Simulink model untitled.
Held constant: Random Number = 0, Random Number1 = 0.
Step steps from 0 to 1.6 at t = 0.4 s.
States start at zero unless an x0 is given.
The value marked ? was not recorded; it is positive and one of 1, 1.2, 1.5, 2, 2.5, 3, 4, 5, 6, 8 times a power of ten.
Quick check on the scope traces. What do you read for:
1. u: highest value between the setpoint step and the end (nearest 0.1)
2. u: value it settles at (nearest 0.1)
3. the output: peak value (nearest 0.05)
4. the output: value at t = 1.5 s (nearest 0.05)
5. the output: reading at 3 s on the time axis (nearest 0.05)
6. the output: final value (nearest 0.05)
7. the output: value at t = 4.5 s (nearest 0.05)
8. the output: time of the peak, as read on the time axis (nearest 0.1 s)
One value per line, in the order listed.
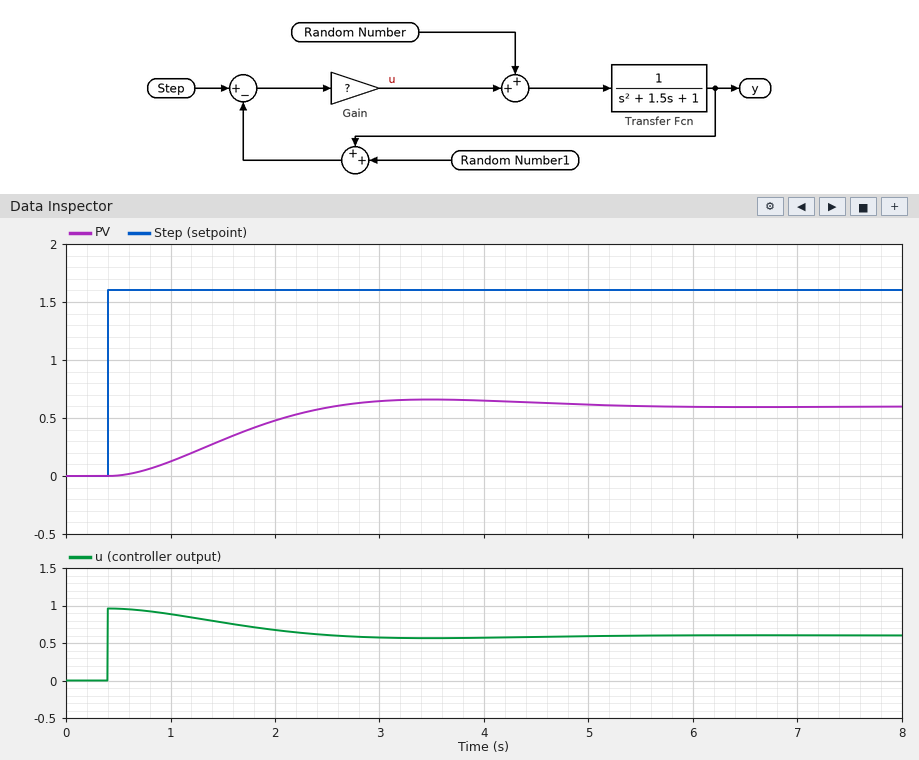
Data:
1.0
0.6
0.65
0.30
0.65
0.60
0.65
3.5 s
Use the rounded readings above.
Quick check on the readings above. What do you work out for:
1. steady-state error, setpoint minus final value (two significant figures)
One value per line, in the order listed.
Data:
1.0
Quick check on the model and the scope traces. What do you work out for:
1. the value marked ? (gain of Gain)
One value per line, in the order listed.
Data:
0.6
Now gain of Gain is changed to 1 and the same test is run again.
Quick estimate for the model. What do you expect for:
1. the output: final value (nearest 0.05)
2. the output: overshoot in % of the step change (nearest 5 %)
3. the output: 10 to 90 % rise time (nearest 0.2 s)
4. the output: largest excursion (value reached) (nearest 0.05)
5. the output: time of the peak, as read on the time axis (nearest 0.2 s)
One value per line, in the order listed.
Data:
0.80
15 %
1.2 s
0.90
3.0 s
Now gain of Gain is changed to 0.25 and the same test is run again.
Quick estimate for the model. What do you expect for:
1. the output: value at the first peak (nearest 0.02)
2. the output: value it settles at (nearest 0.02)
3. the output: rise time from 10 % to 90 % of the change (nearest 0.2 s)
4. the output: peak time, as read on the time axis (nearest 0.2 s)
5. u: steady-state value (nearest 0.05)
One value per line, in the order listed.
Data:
0.34
0.32
1.8 s
4.2 s
0.30
